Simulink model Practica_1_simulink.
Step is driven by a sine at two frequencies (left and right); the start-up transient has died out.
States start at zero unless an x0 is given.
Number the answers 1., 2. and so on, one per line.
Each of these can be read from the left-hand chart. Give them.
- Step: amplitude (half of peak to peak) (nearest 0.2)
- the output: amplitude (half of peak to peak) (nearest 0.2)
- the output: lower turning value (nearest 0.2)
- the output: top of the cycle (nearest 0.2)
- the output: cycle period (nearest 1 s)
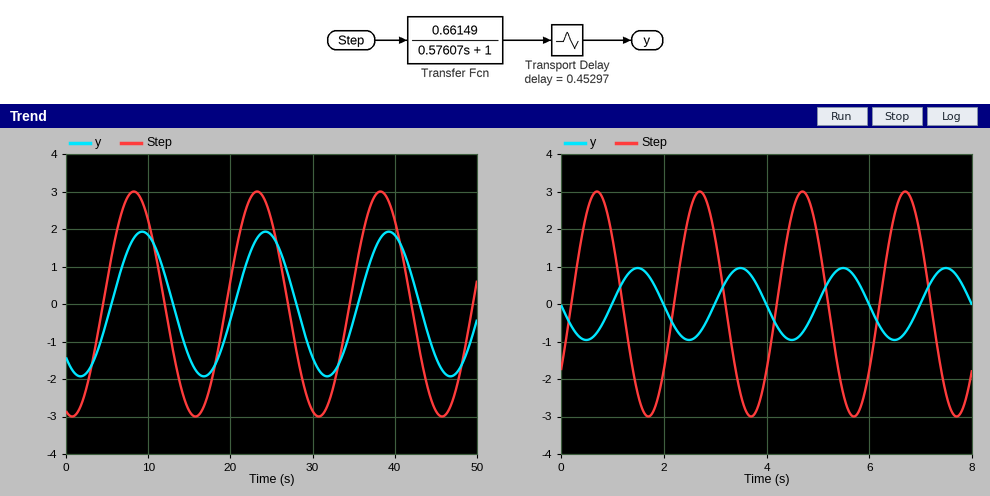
1. 3.0
2. 2.0
3. -2.0
4. 2.0
5. 15 s
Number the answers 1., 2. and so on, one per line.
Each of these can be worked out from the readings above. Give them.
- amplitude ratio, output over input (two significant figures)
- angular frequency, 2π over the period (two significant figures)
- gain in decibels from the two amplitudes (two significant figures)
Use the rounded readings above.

1. 0.67
2. 0.42 rad/s
3. -3.5 dB
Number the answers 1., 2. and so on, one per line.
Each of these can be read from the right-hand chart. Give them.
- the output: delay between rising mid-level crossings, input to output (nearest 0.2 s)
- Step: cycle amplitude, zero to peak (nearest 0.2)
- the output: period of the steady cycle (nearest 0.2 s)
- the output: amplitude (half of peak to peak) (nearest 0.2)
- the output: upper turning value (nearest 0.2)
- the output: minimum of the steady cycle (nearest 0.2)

1. 0.8 s
2. 3.0
3. 2.0 s
4. 1.0
5. 1.0
6. -1.0
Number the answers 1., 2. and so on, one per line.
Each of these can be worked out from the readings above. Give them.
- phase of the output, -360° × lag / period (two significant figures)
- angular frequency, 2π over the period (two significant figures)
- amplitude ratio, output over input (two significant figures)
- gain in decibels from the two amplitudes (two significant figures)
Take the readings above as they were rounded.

1. -140°
2. 3.1 rad/s
3. 0.33
4. -9.5 dB
